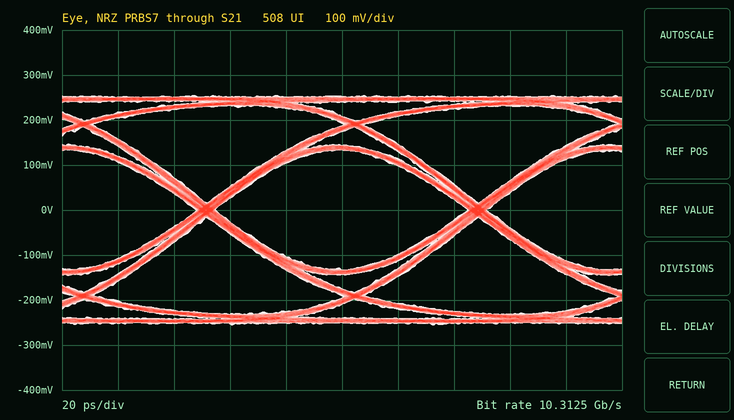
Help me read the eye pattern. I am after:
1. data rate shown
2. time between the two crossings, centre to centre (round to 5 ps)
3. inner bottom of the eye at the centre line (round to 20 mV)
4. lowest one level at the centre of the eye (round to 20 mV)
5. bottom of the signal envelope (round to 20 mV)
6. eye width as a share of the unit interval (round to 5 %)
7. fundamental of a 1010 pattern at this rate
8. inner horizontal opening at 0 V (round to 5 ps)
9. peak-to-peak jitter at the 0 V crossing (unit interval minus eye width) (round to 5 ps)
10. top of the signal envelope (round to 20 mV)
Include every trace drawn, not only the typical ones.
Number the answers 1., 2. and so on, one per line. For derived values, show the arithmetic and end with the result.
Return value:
1. 10.3125 Gb/s
2. 95 ps
3. -140 mV
4. 140 mV
5. -260 mV
6. 90 ps / 95 ps ≈ 95 %
7. 5.15625 GHz
8. 90 ps
9. 5 ps
10. 260 mV
